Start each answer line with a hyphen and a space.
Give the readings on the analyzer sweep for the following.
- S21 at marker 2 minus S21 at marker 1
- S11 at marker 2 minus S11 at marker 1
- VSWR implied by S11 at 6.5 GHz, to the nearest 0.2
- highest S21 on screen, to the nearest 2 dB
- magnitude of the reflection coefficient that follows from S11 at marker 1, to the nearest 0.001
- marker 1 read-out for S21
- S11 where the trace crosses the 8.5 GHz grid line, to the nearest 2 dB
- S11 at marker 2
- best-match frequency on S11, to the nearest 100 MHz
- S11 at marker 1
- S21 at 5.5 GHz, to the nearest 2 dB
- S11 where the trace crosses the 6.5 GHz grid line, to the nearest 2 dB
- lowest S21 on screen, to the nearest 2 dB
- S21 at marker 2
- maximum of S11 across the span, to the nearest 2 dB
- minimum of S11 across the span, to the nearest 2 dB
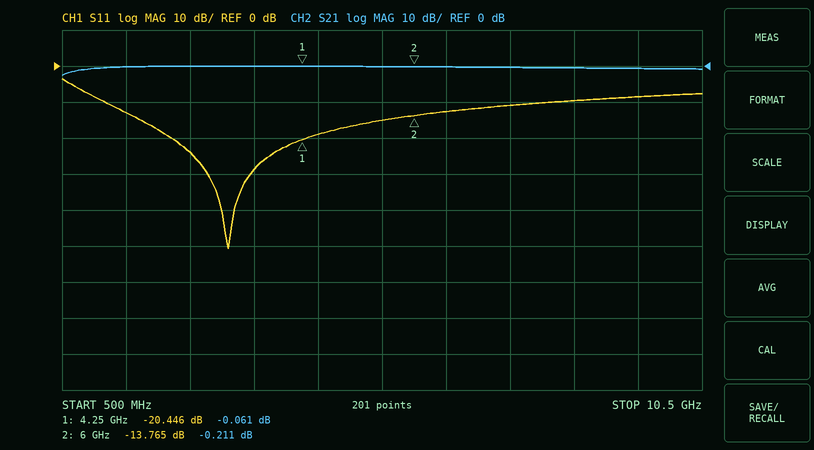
- -0.150 dB
- 6.681 dB
- 1.6
- 0 dB
- 0.095
- -0.061 dB
- -10 dB
- -13.765 dB
- 3.1 GHz
- -20.446 dB
- 0 dB
- -12 dB
- -2 dB
- -0.211 dB
- -4 dB
- -50 dB
